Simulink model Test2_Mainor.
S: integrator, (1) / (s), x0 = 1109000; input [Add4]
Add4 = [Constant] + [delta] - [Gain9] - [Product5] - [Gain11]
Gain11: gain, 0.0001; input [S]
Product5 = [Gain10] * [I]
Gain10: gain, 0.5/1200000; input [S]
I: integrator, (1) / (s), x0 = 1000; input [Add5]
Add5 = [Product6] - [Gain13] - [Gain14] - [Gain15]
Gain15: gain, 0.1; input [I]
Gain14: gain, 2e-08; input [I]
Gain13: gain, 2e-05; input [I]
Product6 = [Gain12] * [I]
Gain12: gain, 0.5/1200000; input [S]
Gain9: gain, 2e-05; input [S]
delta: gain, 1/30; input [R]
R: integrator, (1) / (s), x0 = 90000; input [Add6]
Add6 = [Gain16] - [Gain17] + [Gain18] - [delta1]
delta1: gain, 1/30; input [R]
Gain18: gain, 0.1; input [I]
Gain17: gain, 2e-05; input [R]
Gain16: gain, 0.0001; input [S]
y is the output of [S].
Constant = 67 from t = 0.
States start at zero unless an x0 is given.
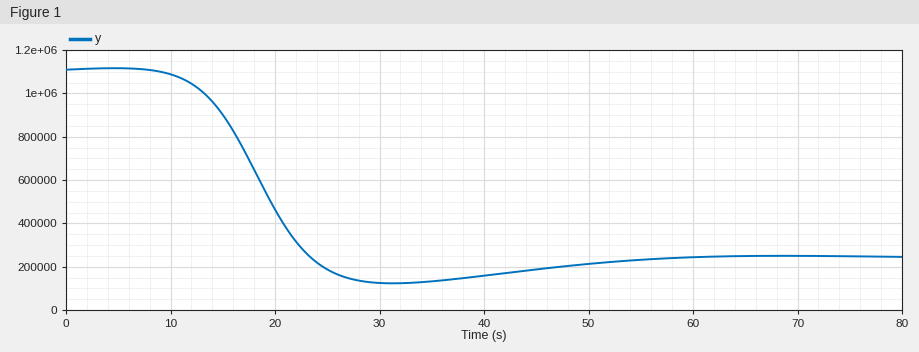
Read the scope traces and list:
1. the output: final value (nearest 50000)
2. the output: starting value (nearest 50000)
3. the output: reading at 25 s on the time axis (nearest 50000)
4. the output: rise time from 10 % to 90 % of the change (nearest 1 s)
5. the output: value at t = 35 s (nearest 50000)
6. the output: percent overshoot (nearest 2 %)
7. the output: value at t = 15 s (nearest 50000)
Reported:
250000
1100000
200000
9 s
150000
14 %
900000
